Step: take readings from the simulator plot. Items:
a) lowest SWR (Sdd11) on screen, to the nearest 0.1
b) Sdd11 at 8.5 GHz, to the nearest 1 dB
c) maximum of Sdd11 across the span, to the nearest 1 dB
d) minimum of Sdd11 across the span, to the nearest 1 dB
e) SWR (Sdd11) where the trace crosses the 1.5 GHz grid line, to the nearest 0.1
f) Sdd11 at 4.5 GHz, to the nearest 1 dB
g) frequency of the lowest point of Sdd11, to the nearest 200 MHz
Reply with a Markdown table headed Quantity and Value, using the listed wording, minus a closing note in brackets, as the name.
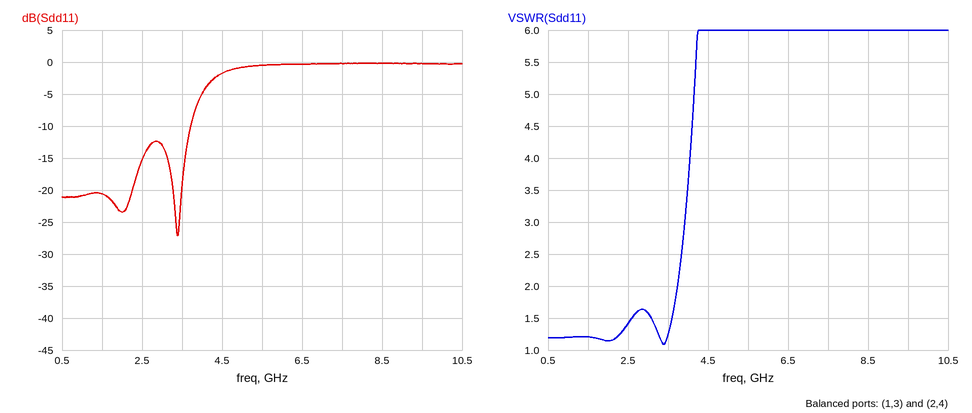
| Quantity | Value |
|---|---|
| lowest SWR (Sdd11) on screen, to the nearest 0.1 | 1.1 |
| Sdd11 at 8.5 GHz, to the nearest 1 dB | 0 dB |
| maximum of Sdd11 across the span, to the nearest 1 dB | 0 dB |
| minimum of Sdd11 across the span, to the nearest 1 dB | -27 dB |
| SWR (Sdd11) where the trace crosses the 1.5 GHz grid line, to the nearest 0.1 | 1.2 |
| Sdd11 at 4.5 GHz, to the nearest 1 dB | -2 dB |
| frequency of the lowest point of Sdd11, to the nearest 200 MHz | 3.4 GHz |
